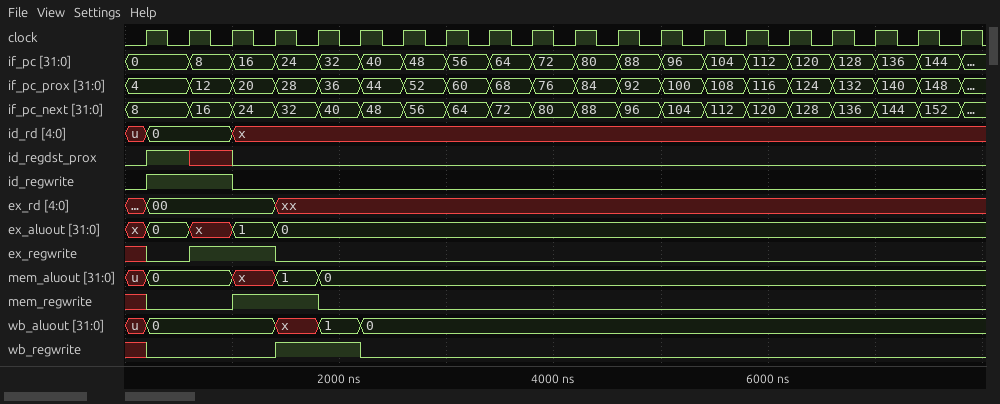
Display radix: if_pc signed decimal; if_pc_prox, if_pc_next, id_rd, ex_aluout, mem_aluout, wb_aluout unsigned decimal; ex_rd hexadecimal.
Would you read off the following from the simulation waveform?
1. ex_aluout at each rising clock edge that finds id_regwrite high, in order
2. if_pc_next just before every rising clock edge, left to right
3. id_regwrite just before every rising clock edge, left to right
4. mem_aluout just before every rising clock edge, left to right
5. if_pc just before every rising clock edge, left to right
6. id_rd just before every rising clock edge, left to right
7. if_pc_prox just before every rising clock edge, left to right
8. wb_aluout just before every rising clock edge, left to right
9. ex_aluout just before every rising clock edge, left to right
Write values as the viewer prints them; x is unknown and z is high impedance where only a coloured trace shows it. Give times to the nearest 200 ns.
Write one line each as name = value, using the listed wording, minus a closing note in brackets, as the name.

ex_aluout at each rising clock edge that finds id_regwrite high, in order = 0, x
if_pc_next just before every rising clock edge, left to right = 8, 8, 16, 24, 32, 40, 48, 56, 64, 72, 80, 88, 96, 104, 112, 120, 128, 136, 144, 152
id_regwrite just before every rising clock edge, left to right = 0 1 1 0 0 0 0 0 0 0 0 0 0 0 0 0 0 0 0 0
mem_aluout just before every rising clock edge, left to right = u, 0, 0, x, 1, 0, 0, 0, 0, 0, 0, 0, 0, 0, 0, 0, 0, 0, 0, 0
if_pc just before every rising clock edge, left to right = 0, 0, 8, 16, 24, 32, 40, 48, 56, 64, 72, 80, 88, 96, 104, 112, 120, 128, 136, 144
id_rd just before every rising clock edge, left to right = u, 0, 0, x, x, x, x, x, x, x, x, x, x, x, x, x, x, x, x, x
if_pc_prox just before every rising clock edge, left to right = 4, 4, 12, 20, 28, 36, 44, 52, 60, 68, 76, 84, 92, 100, 108, 116, 124, 132, 140, 148
wb_aluout just before every rising clock edge, left to right = u, 0, 0, 0, x, 1, 0, 0, 0, 0, 0, 0, 0, 0, 0, 0, 0, 0, 0, 0
ex_aluout just before every rising clock edge, left to right = x, 0, x, 1, 0, 0, 0, 0, 0, 0, 0, 0, 0, 0, 0, 0, 0, 0, 0, 0
